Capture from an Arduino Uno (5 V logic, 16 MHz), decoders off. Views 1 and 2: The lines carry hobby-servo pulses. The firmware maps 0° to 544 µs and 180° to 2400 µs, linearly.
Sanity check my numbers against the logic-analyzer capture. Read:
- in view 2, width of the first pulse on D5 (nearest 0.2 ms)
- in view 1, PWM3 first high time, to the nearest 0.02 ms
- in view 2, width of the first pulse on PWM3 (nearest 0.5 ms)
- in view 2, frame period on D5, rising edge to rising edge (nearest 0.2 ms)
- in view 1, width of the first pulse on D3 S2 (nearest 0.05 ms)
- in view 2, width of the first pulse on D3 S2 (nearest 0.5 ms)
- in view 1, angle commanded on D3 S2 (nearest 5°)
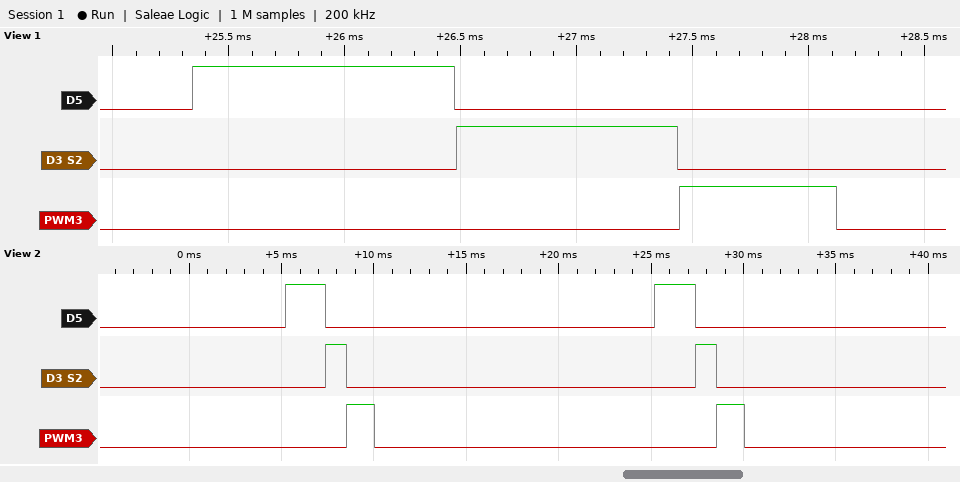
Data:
2.2 ms
0.68 ms
1.5 ms
20.0 ms
0.95 ms
1.0 ms
40°
